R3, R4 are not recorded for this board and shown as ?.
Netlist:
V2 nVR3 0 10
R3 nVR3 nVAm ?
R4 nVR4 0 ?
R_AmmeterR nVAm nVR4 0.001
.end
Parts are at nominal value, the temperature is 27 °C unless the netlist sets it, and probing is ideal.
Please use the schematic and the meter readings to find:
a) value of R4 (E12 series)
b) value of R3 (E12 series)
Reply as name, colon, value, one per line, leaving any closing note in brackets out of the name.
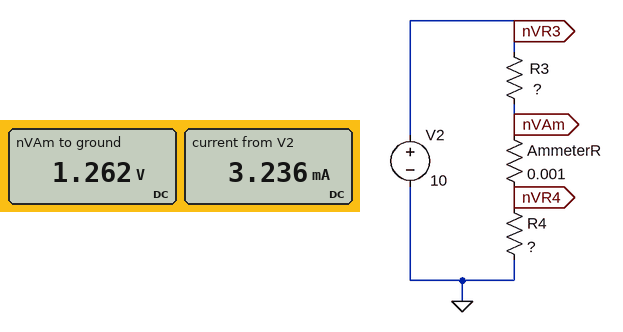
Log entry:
value of R4: 390 Ω
value of R3: 2.7 kΩ
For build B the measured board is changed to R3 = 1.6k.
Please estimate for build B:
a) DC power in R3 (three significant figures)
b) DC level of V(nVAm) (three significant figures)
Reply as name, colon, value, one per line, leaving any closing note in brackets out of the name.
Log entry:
DC power in R3: 40.4 mW
DC level of V(nVAm): 1.96 V
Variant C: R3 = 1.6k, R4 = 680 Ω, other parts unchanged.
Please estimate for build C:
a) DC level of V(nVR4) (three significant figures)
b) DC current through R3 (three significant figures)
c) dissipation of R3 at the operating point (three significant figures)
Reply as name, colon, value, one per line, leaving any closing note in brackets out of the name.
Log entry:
DC level of V(nVR4): 2.98 V
DC current through R3: 4.39 mA
dissipation of R3 at the operating point: 30.8 mW
